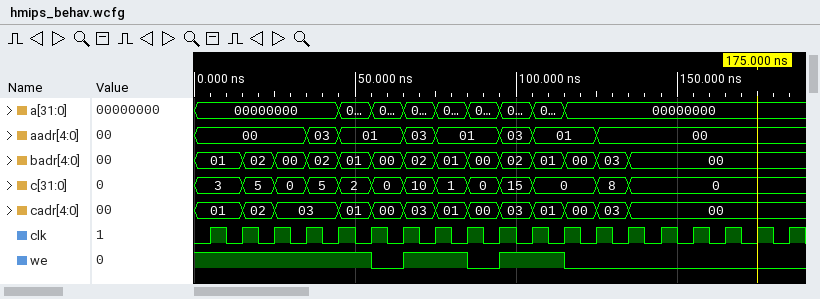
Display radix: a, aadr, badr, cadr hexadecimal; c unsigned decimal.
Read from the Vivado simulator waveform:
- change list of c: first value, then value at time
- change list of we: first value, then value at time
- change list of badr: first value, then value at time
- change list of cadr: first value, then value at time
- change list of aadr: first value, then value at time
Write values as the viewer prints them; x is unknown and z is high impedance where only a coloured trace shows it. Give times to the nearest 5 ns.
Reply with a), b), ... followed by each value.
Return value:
a) 3, 5 at 15 ns, 0 at 25 ns, 5 at 35 ns, 2 at 45 ns, 0 at 55 ns, 10 at 65 ns, 1 at 75 ns, 0 at 85 ns, 15 at 95 ns, 0 at 105 ns, 8 at 125 ns, 0 at 135 ns
b) 1, 0 at 55 ns, 1 at 65 ns, 0 at 85 ns, 1 at 95 ns, 0 at 115 ns
c) 01, 02 at 15 ns, 00 at 25 ns, 02 at 35 ns, 01 at 45 ns, 00 at 55 ns, 02 at 65 ns, 01 at 75 ns, 00 at 85 ns, 02 at 95 ns, 01 at 105 ns, 00 at 115 ns, 03 at 125 ns, 00 at 135 ns
d) 01, 02 at 15 ns, 03 at 25 ns, 01 at 45 ns, 00 at 55 ns, 03 at 65 ns, 01 at 75 ns, 00 at 85 ns, 03 at 95 ns, 01 at 105 ns, 00 at 115 ns, 03 at 125 ns, 00 at 135 ns
e) 00, 03 at 35 ns, 01 at 45 ns, 03 at 65 ns, 01 at 75 ns, 03 at 95 ns, 01 at 105 ns, 00 at 125 ns
